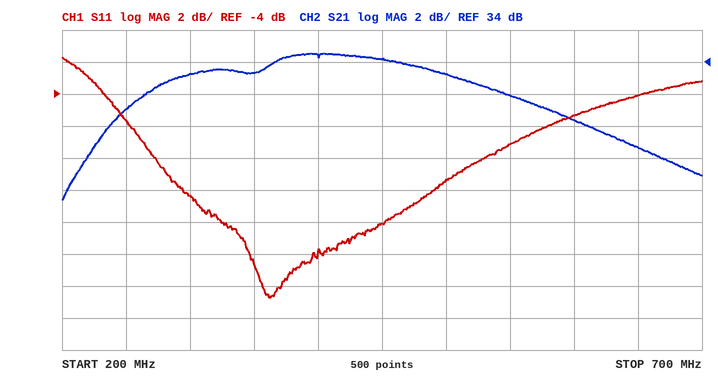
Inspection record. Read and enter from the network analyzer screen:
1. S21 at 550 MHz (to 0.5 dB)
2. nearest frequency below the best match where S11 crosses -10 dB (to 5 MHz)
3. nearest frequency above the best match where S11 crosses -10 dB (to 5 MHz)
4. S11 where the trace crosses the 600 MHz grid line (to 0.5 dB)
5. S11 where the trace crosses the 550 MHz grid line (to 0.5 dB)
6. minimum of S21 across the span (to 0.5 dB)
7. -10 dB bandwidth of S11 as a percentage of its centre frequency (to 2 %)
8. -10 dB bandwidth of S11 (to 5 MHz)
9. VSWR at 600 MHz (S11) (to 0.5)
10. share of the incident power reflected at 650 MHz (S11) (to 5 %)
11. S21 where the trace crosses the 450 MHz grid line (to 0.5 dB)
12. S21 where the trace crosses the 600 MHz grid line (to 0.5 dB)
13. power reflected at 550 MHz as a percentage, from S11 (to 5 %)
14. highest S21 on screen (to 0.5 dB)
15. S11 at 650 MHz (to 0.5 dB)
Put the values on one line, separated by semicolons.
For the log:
32.0 dB; 295 MHz; 490 MHz; -5.5 dB; -7.0 dB; 25.5 dB; 50 %; 195 MHz; 3.5; 40 %; 34.0 dB; 30.5 dB; 20 %; 34.5 dB; -4.0 dB
